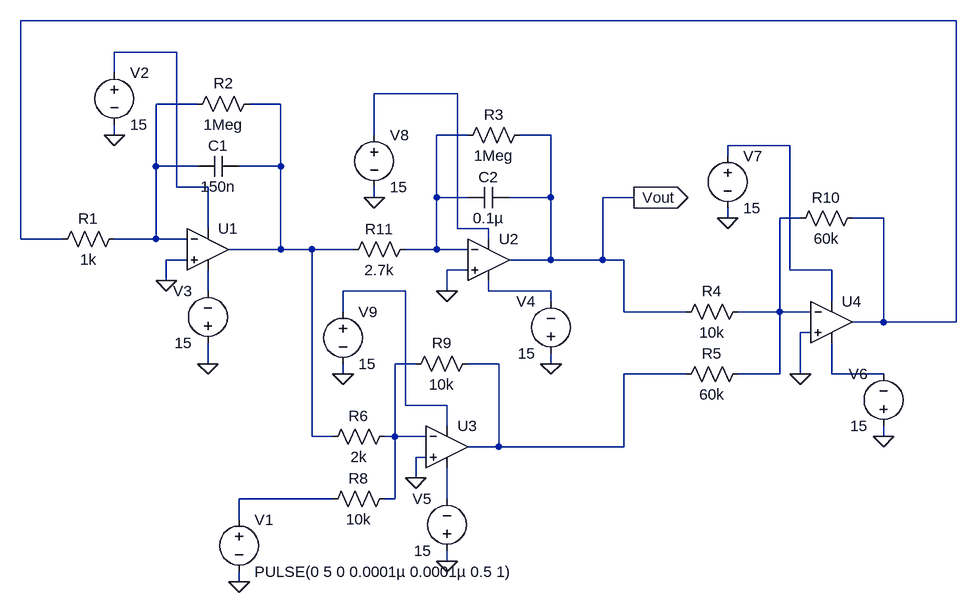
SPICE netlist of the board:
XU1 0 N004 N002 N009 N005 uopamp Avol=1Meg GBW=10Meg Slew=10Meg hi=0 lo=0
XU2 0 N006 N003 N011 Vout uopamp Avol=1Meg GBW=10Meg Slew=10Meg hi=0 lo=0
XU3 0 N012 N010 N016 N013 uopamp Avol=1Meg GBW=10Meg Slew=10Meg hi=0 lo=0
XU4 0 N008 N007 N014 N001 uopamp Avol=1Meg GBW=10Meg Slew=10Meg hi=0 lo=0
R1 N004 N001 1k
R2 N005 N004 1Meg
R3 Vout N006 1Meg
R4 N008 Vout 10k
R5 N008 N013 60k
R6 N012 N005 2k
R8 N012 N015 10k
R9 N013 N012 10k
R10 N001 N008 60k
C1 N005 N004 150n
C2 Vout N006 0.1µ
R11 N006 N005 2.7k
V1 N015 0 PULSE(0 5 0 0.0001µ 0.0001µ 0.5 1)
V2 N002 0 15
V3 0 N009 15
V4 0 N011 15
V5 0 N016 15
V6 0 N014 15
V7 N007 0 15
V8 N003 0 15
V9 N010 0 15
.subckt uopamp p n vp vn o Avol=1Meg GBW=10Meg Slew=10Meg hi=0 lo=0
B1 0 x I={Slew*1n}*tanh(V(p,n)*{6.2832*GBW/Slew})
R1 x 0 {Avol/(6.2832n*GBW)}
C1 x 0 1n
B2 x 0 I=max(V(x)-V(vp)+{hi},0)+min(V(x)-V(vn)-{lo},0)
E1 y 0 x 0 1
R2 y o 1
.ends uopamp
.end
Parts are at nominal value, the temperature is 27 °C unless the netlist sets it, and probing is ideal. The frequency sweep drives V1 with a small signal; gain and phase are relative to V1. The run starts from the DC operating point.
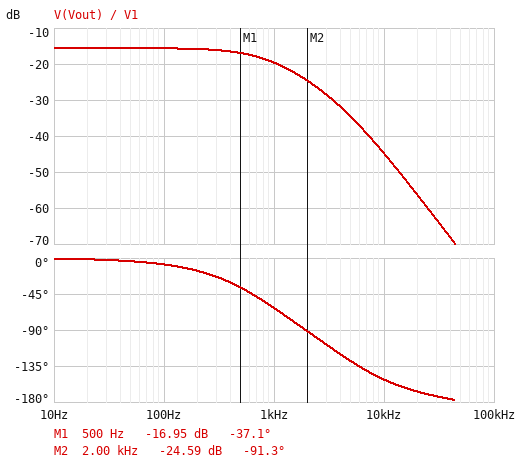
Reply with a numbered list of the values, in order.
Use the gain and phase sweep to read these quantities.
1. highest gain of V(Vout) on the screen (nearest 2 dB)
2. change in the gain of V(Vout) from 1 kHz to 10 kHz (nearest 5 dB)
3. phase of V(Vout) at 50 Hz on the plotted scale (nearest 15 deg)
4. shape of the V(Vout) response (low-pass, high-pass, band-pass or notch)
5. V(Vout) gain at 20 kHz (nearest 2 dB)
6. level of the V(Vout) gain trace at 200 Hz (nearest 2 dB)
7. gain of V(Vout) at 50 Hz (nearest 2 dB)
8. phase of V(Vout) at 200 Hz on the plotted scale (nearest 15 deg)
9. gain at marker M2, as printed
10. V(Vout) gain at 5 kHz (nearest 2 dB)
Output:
1. -16 dB
2. -25 dB
3. 0 deg
4. low-pass
5. -56 dB
6. -16 dB
7. -16 dB
8. -15 deg
9. -24.59 dB
10. -34 dB
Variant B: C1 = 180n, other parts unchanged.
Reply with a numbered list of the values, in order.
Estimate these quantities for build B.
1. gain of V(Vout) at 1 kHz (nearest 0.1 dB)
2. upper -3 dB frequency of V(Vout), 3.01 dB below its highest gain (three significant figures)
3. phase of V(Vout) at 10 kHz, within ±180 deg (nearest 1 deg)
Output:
1. -19.5 dB
2. 837 Hz
3. -156 deg
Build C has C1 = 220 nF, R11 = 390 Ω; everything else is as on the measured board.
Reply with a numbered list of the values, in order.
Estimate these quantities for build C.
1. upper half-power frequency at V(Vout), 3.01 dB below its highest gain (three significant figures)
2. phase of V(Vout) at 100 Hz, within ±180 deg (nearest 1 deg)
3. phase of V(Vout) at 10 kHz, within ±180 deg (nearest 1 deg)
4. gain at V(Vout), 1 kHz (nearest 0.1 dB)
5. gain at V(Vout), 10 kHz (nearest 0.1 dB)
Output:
1. 5.01 kHz
2. -1 deg
3. -157 deg
4. -15.3 dB
5. -29.6 dB
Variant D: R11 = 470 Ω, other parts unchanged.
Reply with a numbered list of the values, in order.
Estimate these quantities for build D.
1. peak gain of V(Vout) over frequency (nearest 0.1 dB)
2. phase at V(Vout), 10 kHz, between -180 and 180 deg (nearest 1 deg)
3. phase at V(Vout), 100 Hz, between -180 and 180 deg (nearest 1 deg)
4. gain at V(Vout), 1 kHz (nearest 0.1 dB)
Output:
1. -15.0 dB
2. -147 deg
3. -1 deg
4. -15.4 dB
